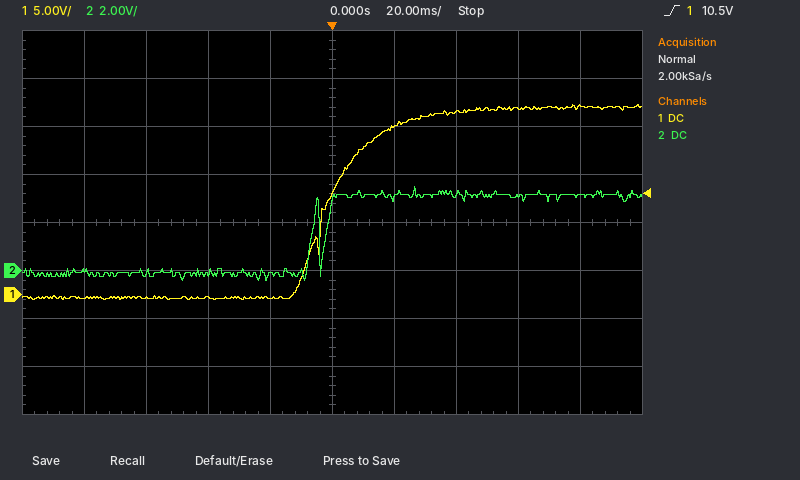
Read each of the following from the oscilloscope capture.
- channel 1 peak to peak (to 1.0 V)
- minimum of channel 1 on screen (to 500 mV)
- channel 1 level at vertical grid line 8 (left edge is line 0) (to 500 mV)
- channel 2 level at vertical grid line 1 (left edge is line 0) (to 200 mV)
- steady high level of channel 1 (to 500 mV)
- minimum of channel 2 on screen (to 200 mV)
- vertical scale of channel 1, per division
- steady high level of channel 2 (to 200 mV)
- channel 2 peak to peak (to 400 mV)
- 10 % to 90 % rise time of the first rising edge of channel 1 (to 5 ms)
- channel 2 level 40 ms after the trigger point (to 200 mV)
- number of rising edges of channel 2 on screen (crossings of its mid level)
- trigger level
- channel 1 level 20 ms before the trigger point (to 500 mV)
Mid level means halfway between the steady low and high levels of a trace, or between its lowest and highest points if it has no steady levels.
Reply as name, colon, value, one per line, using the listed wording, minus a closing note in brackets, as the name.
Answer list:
channel 1 peak to peak: 20.0 V
minimum of channel 1 on screen: -500 mV
channel 1 level at vertical grid line 8 (left edge is line 0): 19.5 V
channel 2 level at vertical grid line 1 (left edge is line 0): 0.0 V
steady high level of channel 1: 19.5 V
minimum of channel 2 on screen: -400 mV
vertical scale of channel 1, per division: 5 V
steady high level of channel 2: 3.2 V
channel 2 peak to peak: 4.0 V
10 % to 90 % rise time of the first rising edge of channel 1: 30 ms
channel 2 level 40 ms after the trigger point: 3.2 V
number of rising edges of channel 2 on screen: 2
trigger level: 10.5 V
channel 1 level 20 ms before the trigger point: -500 mV
